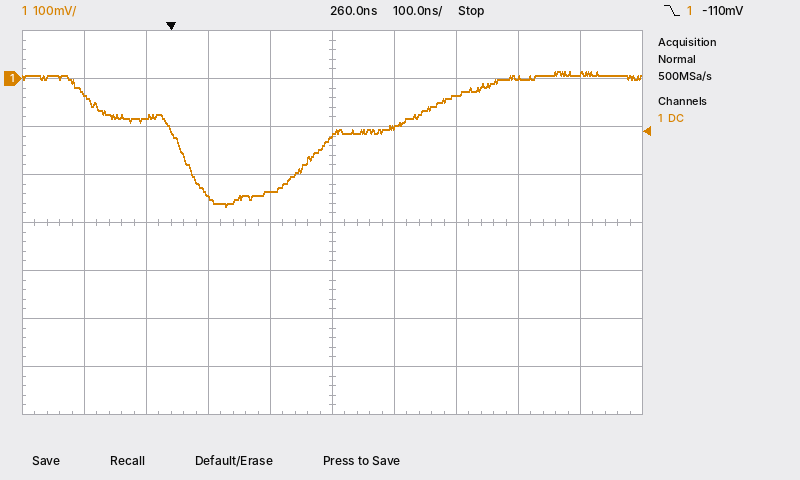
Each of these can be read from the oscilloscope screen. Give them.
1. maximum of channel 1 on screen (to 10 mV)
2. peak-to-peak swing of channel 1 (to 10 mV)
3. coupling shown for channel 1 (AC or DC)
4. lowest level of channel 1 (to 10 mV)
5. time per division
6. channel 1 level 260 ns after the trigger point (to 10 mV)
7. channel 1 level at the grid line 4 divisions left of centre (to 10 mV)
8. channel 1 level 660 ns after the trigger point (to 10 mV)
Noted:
10 mV
280 mV
DC
-270 mV
100 ns
-120 mV
-30 mV
10 mV
